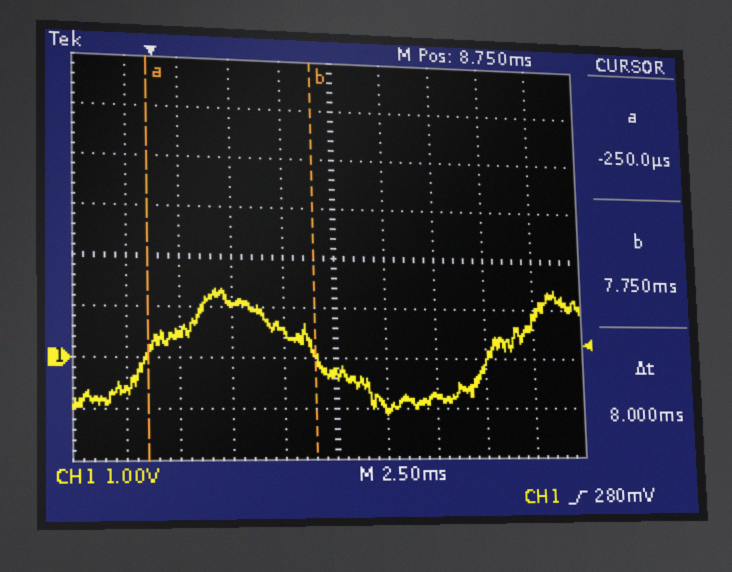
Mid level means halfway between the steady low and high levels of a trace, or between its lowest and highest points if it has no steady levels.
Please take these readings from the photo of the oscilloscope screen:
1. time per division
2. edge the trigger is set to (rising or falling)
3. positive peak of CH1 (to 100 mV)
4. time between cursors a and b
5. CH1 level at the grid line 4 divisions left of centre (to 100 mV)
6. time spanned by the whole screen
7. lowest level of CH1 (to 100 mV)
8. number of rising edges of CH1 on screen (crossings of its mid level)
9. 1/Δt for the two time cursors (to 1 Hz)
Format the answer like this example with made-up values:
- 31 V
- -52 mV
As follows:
- 2.5 ms
- rising
- 1.4 V
- 8 ms
- -600 mV
- 25 ms
- -1.1 V
- 2
- 125 Hz
